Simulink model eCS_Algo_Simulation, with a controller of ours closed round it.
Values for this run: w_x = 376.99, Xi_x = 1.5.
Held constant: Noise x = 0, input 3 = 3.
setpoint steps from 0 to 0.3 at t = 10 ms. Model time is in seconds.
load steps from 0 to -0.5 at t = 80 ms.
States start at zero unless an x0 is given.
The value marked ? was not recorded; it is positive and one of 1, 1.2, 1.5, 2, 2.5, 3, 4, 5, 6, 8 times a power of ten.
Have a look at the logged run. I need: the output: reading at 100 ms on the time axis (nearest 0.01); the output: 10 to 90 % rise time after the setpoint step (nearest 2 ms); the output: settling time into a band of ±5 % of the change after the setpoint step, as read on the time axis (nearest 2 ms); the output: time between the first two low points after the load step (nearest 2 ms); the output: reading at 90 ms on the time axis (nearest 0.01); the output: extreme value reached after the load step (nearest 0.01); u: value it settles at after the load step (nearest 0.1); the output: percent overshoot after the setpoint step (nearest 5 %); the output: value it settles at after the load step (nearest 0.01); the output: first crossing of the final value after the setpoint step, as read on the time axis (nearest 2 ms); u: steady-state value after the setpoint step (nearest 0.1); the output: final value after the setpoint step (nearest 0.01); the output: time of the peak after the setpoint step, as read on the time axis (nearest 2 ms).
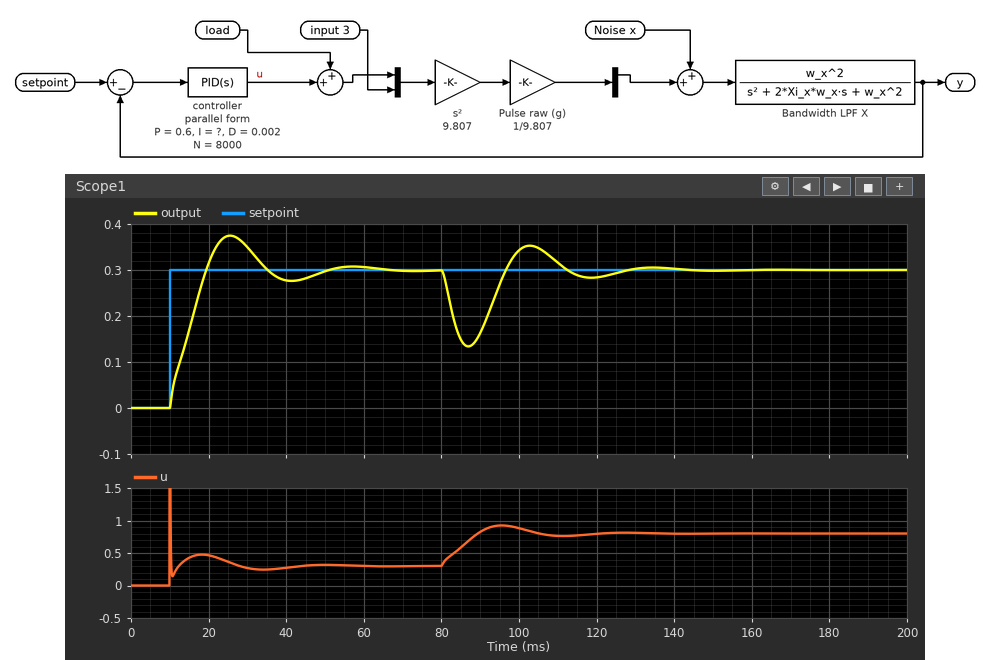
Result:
0.34
8 ms
46 ms
32 ms
0.16
0.13
0.8
25 %
0.30
20 ms
0.3
0.30
26 ms
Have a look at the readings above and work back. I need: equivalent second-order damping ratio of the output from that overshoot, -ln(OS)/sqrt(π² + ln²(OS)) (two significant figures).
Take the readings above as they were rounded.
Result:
0.40
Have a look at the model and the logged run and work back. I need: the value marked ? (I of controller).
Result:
400
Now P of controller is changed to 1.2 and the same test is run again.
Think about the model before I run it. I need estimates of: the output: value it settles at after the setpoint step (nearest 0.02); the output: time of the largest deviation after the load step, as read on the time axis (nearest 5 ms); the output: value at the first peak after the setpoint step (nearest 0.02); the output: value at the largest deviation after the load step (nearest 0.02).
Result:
0.30
85 ms
0.34
0.16
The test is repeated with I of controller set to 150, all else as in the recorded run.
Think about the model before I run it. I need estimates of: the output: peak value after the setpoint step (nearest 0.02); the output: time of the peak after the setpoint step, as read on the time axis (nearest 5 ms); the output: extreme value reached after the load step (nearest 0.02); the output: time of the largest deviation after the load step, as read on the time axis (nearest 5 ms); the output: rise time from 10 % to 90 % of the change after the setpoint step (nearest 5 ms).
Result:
0.32
40 ms
0.10
90 ms
15 ms
